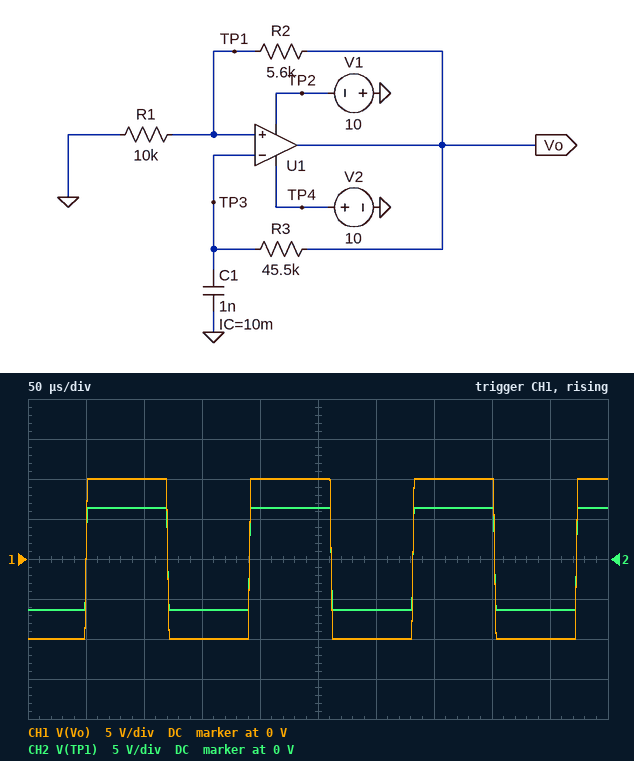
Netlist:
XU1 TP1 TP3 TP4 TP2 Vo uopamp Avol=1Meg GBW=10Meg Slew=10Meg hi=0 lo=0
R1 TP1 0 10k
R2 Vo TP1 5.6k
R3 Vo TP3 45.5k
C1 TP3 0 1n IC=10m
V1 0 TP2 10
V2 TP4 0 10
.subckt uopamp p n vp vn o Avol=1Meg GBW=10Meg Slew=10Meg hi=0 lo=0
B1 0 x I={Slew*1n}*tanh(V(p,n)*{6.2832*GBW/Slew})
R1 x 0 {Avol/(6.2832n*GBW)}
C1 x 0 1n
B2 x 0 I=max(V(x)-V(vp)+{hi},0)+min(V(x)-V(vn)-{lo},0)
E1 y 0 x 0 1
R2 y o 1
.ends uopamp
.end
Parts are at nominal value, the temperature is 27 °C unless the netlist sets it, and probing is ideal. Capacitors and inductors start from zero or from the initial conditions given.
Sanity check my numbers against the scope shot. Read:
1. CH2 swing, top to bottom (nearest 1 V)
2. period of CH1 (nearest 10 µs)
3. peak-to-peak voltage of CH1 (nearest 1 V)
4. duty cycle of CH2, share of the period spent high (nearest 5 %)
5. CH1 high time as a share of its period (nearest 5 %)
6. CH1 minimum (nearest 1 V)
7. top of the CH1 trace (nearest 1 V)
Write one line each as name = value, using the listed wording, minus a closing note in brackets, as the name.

CH2 swing, top to bottom = 13 V
period of CH1 = 140 µs
peak-to-peak voltage of CH1 = 20 V
duty cycle of CH2, share of the period spent high = 50 %
CH1 high time as a share of its period = 50 %
CH1 minimum = -10 V
top of the CH1 trace = 10 V
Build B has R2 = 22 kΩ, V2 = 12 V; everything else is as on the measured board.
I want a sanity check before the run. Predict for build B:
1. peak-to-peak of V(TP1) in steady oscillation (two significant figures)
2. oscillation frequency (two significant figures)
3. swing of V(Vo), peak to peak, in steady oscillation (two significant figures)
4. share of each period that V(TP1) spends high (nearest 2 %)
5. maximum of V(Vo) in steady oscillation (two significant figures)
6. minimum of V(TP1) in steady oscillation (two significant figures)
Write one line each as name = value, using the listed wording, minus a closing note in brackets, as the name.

peak-to-peak of V(TP1) in steady oscillation = 6.9 V
oscillation frequency = 16 kHz
swing of V(Vo), peak to peak, in steady oscillation = 22 V
share of each period that V(TP1) spends high = 46 %
maximum of V(Vo) in steady oscillation = 12 V
minimum of V(TP1) in steady oscillation = -3.1 V
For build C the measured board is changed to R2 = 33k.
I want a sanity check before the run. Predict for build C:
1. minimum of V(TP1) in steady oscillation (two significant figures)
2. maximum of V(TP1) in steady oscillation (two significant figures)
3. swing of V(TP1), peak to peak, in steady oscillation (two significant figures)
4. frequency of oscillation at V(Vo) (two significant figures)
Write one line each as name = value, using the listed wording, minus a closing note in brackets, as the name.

minimum of V(TP1) in steady oscillation = -2.3 V
maximum of V(TP1) in steady oscillation = 2.3 V
swing of V(TP1), peak to peak, in steady oscillation = 4.7 V
frequency of oscillation at V(Vo) = 21 kHz
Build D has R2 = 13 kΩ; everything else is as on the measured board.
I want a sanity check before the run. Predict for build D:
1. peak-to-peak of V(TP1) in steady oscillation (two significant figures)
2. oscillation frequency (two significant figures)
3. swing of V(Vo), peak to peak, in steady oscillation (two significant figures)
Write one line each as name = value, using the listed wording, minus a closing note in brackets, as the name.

peak-to-peak of V(TP1) in steady oscillation = 8.7 V
oscillation frequency = 11 kHz
swing of V(Vo), peak to peak, in steady oscillation = 20 V
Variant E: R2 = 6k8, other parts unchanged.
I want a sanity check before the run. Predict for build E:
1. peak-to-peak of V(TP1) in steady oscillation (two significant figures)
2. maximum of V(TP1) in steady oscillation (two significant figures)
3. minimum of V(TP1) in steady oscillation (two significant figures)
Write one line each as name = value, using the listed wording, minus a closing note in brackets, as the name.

peak-to-peak of V(TP1) in steady oscillation = 12 V
maximum of V(TP1) in steady oscillation = 6.0 V
minimum of V(TP1) in steady oscillation = -6.0 V
